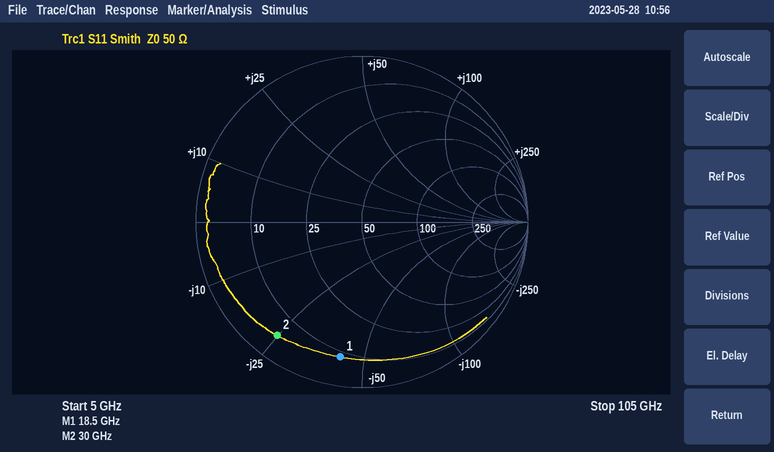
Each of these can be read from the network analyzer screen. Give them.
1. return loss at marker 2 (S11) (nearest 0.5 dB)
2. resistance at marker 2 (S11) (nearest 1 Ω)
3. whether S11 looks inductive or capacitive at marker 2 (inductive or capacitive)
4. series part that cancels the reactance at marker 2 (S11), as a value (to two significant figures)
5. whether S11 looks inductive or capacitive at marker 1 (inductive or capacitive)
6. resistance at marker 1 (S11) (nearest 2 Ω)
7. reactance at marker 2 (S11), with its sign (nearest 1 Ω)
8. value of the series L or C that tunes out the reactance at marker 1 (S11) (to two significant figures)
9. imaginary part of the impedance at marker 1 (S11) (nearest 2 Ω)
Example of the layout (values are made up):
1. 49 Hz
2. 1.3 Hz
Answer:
1. 1.5 dB
2. 5 Ω
3. capacitive
4. 130 pH
5. capacitive
6. 8 Ω
7. -25 Ω
8. 360 pH
9. -42 Ω
